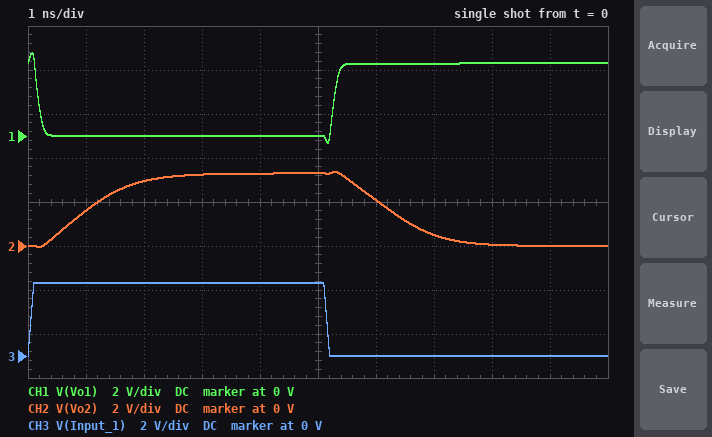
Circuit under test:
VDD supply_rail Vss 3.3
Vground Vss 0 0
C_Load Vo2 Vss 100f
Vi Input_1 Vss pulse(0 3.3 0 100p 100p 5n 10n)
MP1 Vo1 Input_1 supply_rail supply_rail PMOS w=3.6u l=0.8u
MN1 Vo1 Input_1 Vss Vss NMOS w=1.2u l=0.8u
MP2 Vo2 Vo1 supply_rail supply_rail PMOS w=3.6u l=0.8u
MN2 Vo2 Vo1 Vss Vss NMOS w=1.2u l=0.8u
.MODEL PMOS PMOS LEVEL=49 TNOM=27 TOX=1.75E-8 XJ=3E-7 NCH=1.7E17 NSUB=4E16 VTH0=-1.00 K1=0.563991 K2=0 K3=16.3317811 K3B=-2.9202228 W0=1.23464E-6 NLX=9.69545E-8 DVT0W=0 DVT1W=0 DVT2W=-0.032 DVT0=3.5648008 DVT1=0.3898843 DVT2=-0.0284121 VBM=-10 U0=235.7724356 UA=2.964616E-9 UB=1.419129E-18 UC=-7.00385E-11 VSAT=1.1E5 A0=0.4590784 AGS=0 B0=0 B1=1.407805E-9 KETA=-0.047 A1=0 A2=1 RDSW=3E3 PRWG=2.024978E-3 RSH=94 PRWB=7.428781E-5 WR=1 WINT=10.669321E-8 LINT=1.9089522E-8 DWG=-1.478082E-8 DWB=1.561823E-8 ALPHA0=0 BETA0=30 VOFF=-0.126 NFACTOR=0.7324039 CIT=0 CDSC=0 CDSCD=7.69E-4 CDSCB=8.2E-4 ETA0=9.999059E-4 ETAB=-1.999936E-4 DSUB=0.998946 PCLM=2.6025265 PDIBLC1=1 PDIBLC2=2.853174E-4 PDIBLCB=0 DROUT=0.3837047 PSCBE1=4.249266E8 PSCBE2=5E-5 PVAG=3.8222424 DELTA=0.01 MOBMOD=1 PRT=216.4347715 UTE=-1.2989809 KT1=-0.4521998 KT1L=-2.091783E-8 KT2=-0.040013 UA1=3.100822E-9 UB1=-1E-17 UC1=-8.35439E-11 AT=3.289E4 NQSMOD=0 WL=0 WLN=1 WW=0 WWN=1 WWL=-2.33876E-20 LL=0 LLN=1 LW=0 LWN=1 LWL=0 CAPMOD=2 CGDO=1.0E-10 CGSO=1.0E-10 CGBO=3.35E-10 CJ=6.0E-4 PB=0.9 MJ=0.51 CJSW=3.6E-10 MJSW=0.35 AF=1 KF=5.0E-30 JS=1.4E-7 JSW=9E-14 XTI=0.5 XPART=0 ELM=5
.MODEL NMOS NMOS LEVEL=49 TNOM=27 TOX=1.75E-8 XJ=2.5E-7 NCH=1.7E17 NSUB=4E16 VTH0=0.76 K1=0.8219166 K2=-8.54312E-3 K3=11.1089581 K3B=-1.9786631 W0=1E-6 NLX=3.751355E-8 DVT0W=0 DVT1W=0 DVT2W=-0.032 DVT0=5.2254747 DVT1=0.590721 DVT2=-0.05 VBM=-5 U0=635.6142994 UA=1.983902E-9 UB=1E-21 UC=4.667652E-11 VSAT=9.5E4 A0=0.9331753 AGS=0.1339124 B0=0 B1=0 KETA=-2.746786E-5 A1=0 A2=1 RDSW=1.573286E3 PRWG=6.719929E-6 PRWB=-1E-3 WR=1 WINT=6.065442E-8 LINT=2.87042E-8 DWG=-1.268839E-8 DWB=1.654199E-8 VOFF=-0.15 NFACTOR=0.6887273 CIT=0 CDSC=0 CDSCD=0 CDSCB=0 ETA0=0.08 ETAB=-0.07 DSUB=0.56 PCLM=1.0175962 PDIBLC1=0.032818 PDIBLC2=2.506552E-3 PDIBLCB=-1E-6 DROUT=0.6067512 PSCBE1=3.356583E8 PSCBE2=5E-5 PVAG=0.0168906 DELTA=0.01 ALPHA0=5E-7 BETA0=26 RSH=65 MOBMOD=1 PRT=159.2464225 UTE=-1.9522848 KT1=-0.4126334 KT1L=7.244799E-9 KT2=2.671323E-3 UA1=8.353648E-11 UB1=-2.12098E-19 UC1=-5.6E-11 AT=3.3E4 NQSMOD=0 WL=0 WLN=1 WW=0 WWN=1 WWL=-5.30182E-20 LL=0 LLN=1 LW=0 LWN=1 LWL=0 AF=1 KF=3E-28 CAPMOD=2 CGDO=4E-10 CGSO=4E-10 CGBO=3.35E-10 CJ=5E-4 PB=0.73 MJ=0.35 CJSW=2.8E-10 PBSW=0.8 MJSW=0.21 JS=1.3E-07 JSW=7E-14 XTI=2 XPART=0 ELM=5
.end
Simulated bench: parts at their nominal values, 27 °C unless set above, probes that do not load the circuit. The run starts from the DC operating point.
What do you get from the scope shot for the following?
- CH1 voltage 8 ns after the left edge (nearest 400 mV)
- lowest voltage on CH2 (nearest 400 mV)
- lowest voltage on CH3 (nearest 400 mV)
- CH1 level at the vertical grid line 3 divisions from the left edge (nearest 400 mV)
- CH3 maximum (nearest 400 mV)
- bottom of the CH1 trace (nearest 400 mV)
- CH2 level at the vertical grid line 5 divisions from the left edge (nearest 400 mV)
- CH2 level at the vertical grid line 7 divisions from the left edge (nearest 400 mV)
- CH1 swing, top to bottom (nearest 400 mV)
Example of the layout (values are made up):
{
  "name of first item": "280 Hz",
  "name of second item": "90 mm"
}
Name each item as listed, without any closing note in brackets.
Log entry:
{
  "CH1 voltage 8 ns after the left edge": "3.2 V",
  "lowest voltage on CH2": "0 V",
  "lowest voltage on CH3": "0 V",
  "CH1 level at the vertical grid line 3 divisions from the left edge": "0 V",
  "CH3 maximum": "3.2 V",
  "bottom of the CH1 trace": "-400 mV",
  "CH2 level at the vertical grid line 5 divisions from the left edge": "3.2 V",
  "CH2 level at the vertical grid line 7 divisions from the left edge": "400 mV",
  "CH1 swing, top to bottom": "4.0 V"
}
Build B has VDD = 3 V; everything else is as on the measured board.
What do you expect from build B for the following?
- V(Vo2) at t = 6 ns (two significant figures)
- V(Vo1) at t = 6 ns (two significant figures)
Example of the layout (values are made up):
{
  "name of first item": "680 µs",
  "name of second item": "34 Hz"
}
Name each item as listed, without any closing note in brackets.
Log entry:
{
  "V(Vo2) at t = 6 ns": "2.0 V",
  "V(Vo1) at t = 6 ns": "3.0 V"
}
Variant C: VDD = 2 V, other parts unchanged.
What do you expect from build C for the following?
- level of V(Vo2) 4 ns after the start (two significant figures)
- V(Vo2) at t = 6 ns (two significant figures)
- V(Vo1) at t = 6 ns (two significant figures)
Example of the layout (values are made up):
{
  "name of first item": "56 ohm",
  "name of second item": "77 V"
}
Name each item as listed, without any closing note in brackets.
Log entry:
{
  "level of V(Vo2) 4 ns after the start": "1.8 V",
  "V(Vo2) at t = 6 ns": "1.7 V",
  "V(Vo1) at t = 6 ns": "2.0 V"
}
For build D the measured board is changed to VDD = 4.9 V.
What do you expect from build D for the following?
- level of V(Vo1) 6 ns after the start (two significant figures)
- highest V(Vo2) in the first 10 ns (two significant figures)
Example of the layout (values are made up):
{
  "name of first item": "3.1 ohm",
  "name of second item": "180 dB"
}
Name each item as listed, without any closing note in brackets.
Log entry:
{
  "level of V(Vo1) 6 ns after the start": "4.9 V",
  "highest V(Vo2) in the first 10 ns": "5.0 V"
}
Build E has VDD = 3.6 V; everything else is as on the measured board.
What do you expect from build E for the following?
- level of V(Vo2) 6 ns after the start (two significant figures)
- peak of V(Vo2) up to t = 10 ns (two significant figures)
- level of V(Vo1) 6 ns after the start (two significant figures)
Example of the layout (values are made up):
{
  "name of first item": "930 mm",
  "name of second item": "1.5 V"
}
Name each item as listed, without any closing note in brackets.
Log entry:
{
  "level of V(Vo2) 6 ns after the start": "2.1 V",
  "peak of V(Vo2) up to t = 10 ns": "3.7 V",
  "level of V(Vo1) 6 ns after the start": "3.6 V"
}
